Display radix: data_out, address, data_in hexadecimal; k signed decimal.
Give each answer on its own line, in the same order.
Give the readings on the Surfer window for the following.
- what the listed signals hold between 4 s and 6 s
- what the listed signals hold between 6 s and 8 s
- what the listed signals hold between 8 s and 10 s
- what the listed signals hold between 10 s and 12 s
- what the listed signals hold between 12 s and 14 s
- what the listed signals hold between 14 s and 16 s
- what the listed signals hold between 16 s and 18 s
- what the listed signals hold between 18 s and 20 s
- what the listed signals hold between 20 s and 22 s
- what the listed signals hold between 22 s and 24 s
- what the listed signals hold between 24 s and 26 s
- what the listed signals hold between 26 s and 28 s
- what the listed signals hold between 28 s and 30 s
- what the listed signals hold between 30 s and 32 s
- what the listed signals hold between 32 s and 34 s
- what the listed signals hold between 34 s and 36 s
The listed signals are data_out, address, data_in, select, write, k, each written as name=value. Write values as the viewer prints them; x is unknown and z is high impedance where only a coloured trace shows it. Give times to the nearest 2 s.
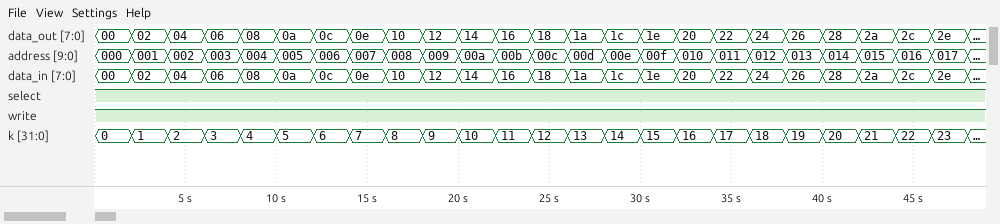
data_out=04, address=002, data_in=04, select=1, write=1, k=2
data_out=06, address=003, data_in=06, select=1, write=1, k=3
data_out=08, address=004, data_in=08, select=1, write=1, k=4
data_out=0a, address=005, data_in=0a, select=1, write=1, k=5
data_out=0c, address=006, data_in=0c, select=1, write=1, k=6
data_out=0e, address=007, data_in=0e, select=1, write=1, k=7
data_out=10, address=008, data_in=10, select=1, write=1, k=8
data_out=12, address=009, data_in=12, select=1, write=1, k=9
data_out=14, address=00a, data_in=14, select=1, write=1, k=10
data_out=16, address=00b, data_in=16, select=1, write=1, k=11
data_out=18, address=00c, data_in=18, select=1, write=1, k=12
data_out=1a, address=00d, data_in=1a, select=1, write=1, k=13
data_out=1c, address=00e, data_in=1c, select=1, write=1, k=14
data_out=1e, address=00f, data_in=1e, select=1, write=1, k=15
data_out=20, address=010, data_in=20, select=1, write=1, k=16
data_out=22, address=011, data_in=22, select=1, write=1, k=17
